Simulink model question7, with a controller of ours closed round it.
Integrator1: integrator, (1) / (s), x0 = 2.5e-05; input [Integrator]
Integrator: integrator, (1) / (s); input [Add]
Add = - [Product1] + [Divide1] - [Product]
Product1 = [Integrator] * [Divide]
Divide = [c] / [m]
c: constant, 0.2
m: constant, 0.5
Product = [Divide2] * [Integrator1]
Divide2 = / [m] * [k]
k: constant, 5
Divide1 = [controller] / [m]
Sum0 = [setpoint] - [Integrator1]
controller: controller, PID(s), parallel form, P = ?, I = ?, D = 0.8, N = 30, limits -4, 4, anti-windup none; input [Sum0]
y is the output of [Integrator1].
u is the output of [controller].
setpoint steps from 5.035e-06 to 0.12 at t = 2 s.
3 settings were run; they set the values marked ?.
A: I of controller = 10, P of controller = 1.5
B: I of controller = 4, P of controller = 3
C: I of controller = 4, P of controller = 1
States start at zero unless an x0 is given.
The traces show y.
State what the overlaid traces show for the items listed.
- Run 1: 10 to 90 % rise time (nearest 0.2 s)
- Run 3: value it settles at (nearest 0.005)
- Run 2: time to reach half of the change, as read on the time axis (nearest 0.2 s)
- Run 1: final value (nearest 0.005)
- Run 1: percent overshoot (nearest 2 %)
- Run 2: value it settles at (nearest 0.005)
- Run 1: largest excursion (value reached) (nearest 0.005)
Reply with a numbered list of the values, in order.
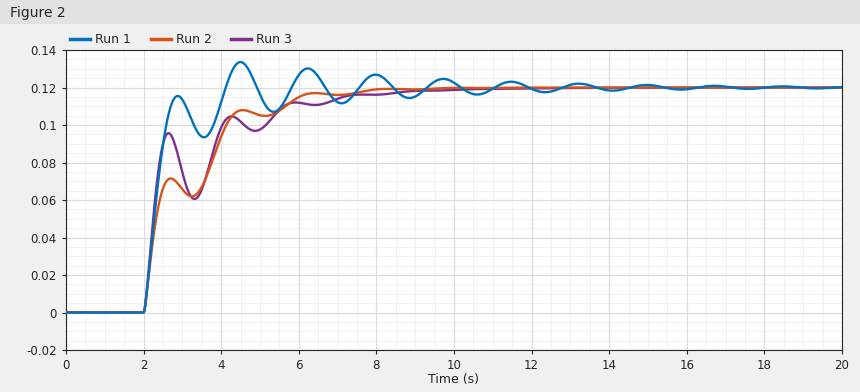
1. 0.6 s
2. 0.120
3. 2.4 s
4. 0.120
5. 12 %
6. 0.120
7. 0.135
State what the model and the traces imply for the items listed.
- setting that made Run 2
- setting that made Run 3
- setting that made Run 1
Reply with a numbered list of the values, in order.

1. C
2. B
3. A
